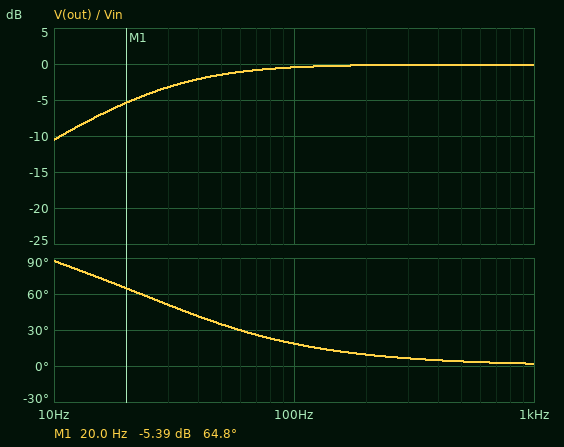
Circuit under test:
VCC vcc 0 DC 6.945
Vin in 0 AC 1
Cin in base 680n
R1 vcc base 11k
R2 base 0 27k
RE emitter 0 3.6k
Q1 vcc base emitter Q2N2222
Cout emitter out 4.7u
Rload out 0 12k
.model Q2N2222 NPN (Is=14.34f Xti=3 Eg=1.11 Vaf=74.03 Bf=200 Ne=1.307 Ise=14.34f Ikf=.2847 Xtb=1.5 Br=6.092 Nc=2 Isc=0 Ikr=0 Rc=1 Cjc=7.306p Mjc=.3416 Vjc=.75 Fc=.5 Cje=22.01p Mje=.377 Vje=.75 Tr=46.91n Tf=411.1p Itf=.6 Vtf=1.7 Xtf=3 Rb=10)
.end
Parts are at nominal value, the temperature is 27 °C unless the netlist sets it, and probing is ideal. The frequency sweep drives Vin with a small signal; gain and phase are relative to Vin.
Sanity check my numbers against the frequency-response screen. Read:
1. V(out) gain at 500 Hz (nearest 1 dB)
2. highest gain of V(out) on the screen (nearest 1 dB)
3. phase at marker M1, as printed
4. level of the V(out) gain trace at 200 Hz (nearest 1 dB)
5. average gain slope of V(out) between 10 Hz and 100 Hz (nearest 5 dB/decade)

0 dB
0 dB
64.8 deg
0 dB
10 dB/decade
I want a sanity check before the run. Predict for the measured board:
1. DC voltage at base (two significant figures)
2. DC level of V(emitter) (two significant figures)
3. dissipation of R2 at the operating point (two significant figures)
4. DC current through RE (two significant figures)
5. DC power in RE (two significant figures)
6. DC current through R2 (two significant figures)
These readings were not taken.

4.9 V
4.2 V
880 µW
1.2 mA
4.9 mW
180 µA
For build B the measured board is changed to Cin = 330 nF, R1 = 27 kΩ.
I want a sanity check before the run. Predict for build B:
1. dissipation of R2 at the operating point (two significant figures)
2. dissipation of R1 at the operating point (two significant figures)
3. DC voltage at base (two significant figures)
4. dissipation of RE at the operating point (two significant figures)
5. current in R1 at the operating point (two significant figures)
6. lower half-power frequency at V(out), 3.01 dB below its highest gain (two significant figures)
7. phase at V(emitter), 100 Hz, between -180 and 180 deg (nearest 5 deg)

430 µW
470 µW
3.4 V
2.1 mW
130 µA
37 Hz
20 deg
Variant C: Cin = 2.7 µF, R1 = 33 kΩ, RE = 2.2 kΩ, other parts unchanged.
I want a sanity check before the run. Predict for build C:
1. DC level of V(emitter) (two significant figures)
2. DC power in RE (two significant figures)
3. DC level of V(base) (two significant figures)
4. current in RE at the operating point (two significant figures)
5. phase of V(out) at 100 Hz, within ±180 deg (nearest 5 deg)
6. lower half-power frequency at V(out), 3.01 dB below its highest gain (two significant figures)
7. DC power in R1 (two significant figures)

2.4 V
2.5 mW
3.0 V
1.1 mA
5 deg
5.5 Hz
470 µW
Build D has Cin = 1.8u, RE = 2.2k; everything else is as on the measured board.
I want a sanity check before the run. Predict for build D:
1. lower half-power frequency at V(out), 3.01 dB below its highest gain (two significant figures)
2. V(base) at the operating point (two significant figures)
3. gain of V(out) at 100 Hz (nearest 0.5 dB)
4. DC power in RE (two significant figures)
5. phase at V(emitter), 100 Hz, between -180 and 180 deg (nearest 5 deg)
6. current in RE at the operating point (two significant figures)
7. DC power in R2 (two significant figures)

12 Hz
4.8 V
0 dB
7.9 mW
5 deg
1.9 mA
860 µW
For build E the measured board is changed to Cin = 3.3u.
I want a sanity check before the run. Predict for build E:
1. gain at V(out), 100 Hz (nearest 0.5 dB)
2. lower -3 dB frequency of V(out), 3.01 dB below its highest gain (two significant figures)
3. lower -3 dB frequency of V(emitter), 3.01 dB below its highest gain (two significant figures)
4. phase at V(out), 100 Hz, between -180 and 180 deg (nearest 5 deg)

0 dB
7.3 Hz
6.3 Hz
5 deg
